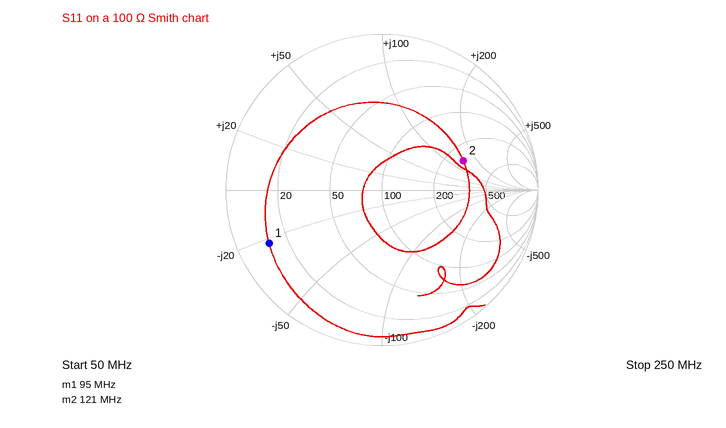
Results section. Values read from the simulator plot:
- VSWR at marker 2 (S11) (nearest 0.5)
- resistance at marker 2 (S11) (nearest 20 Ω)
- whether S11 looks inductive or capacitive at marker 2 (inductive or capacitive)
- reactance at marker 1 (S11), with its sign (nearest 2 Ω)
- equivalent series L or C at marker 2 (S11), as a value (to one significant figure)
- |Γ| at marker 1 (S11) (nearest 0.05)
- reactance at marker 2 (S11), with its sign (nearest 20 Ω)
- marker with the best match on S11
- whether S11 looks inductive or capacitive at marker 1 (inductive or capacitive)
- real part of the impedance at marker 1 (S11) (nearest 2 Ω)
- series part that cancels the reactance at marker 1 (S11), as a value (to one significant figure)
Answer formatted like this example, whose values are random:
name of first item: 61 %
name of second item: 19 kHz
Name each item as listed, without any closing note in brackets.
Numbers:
VSWR at marker 2 (S11): 3.5
resistance at marker 2 (S11): 260 Ω
whether S11 looks inductive or capacitive at marker 2: inductive
reactance at marker 1 (S11), with its sign: -22 Ω
equivalent series L or C at marker 2 (S11), as a value: 200 nH
|Γ| at marker 1 (S11): 0.80
reactance at marker 2 (S11), with its sign: +140 Ω
marker with the best match on S11: marker 2
whether S11 looks inductive or capacitive at marker 1: capacitive
real part of the impedance at marker 1 (S11): 12 Ω
series part that cancels the reactance at marker 1 (S11), as a value: 40 nH
